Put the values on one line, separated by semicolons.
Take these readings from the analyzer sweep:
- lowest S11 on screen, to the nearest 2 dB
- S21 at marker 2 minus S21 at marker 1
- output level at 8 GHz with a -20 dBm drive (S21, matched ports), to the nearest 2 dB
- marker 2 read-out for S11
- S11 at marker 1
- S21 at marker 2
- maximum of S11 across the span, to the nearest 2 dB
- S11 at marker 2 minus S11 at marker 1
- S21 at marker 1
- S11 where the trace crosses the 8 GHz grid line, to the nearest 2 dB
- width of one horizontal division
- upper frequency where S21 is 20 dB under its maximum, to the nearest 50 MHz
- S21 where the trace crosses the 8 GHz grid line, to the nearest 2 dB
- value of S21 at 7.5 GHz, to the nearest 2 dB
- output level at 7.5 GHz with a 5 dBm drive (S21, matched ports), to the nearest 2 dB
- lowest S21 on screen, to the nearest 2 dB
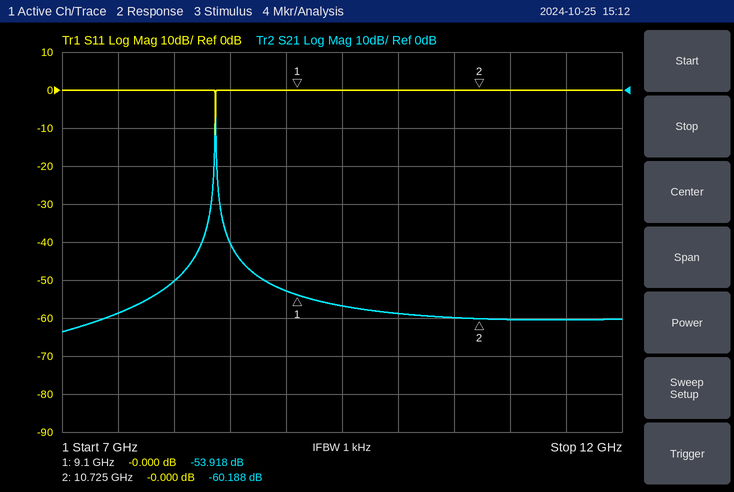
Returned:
-12 dB; -6.270 dB; -70 dBm; -0.000 dB; -0.000 dB; -60.188 dB; 0 dB; 0.000 dB; -53.918 dB; 0 dB; 500 MHz; 8.40 GHz; -50 dB; -58 dB; -54 dBm; -64 dB
